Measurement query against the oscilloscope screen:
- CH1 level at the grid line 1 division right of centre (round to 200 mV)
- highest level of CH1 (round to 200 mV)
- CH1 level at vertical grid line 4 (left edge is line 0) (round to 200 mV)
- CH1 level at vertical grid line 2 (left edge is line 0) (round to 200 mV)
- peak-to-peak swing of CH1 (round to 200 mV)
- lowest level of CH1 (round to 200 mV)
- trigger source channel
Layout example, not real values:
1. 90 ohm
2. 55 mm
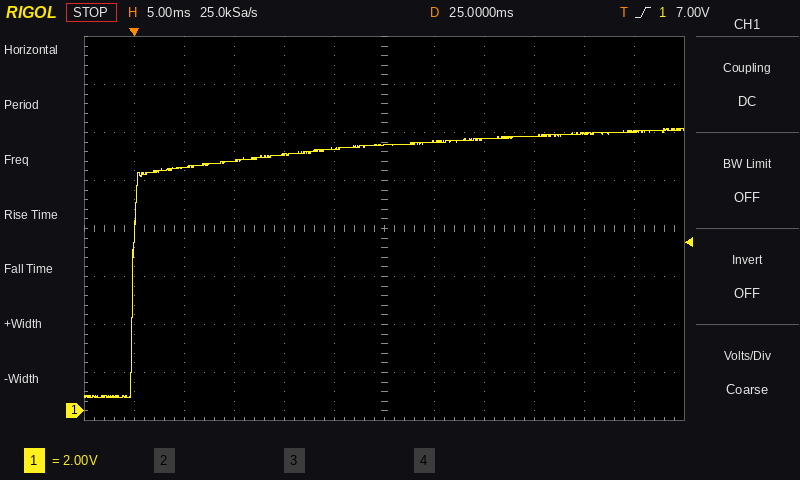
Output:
1. 11.2 V
2. 11.8 V
3. 10.6 V
4. 10.2 V
5. 11.2 V
6. 600 mV
7. CH1
